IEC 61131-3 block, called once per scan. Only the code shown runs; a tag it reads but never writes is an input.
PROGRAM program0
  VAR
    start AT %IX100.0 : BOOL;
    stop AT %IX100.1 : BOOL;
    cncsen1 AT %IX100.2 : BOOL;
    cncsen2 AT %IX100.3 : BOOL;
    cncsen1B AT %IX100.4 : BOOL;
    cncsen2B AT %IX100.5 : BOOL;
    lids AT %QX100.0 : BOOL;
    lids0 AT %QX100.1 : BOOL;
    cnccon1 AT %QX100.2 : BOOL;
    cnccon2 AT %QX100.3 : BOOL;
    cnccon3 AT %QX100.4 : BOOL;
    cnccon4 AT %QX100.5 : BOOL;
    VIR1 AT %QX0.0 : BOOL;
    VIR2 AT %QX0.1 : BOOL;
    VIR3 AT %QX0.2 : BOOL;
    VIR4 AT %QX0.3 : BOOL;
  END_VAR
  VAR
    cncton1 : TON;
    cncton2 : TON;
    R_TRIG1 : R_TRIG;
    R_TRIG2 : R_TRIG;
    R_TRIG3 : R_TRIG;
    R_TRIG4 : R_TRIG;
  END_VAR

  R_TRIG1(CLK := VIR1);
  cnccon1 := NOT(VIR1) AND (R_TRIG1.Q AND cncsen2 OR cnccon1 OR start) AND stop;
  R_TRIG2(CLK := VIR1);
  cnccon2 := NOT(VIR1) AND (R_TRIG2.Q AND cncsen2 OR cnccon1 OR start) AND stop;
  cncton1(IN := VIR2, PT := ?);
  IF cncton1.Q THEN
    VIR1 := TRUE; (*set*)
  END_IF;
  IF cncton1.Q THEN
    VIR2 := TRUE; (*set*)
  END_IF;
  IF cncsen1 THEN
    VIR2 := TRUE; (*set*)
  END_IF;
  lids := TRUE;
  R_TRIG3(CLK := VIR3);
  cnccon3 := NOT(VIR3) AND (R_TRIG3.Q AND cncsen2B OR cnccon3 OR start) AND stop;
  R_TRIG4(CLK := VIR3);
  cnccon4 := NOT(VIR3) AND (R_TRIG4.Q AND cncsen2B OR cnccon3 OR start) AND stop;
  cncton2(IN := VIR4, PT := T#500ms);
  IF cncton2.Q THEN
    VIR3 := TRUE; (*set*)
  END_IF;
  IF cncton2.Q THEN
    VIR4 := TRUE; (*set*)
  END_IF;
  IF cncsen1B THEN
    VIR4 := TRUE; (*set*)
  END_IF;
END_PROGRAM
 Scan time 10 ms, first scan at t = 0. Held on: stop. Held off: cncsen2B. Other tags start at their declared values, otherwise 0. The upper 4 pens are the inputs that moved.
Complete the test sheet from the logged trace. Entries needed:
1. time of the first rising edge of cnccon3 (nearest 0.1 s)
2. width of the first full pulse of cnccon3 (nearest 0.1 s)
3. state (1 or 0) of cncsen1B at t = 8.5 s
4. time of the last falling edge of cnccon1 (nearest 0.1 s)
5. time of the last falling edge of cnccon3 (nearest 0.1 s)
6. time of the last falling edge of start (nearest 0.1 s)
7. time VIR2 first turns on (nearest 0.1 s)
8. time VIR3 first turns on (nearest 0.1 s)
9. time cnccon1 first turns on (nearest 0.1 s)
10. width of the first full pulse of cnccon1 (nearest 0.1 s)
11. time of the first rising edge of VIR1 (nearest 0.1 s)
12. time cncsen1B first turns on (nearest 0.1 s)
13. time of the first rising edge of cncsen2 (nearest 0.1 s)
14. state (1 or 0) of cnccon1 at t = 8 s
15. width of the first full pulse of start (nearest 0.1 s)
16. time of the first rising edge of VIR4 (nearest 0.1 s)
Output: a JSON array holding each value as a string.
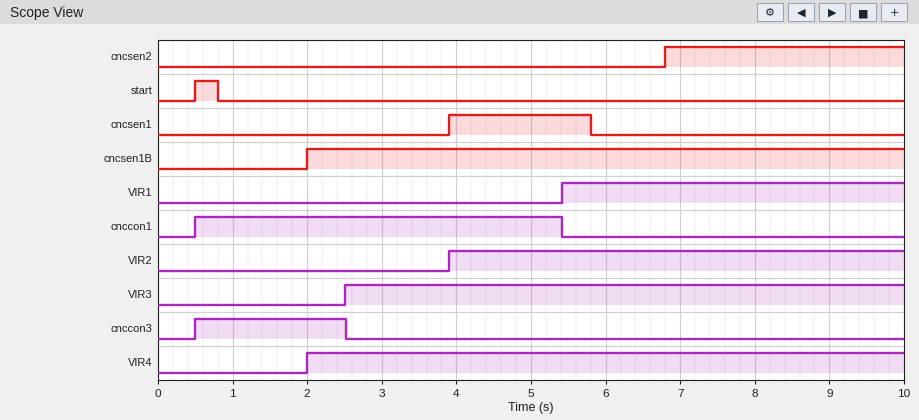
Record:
["0.5 s", "2.0 s", "1", "5.4 s", "2.5 s", "0.8 s", "3.9 s", "2.5 s", "0.5 s", "4.9 s", "5.4 s", "2.0 s", "6.8 s", "0", "0.3 s", "2.0 s"]
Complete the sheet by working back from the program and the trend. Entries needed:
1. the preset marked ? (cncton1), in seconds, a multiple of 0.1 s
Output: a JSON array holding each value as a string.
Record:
["1.5 s"]
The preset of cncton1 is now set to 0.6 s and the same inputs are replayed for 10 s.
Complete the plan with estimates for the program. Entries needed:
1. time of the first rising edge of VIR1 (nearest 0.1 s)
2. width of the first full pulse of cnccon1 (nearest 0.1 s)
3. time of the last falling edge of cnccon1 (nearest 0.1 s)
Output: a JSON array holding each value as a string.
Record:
["4.5 s", "4.0 s", "4.5 s"]
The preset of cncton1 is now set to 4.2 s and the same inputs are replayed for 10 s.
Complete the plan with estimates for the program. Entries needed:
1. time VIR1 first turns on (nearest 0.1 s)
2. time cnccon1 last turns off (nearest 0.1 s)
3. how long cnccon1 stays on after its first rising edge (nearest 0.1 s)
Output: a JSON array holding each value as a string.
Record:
["8.1 s", "8.1 s", "7.6 s"]
